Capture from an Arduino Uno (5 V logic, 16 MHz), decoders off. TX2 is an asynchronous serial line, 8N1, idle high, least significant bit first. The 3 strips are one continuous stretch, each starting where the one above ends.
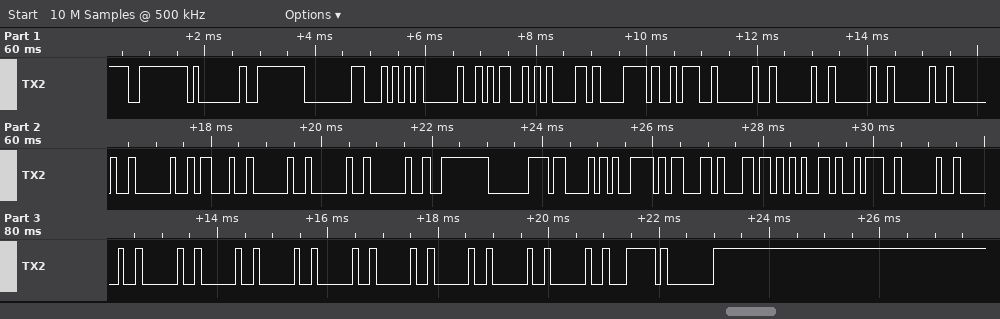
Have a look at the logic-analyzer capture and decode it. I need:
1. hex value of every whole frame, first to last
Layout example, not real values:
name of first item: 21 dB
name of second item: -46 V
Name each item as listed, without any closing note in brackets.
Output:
hex value of every whole frame, first to last: FE 01 FE 80 54 20 4D 61 78 3A 20 20 20 20 20 20 23 20 20 20 FE C0 43 79 63 6C 65 3A 20 20 20 20 20 20 20 20 20 20 7C 80
